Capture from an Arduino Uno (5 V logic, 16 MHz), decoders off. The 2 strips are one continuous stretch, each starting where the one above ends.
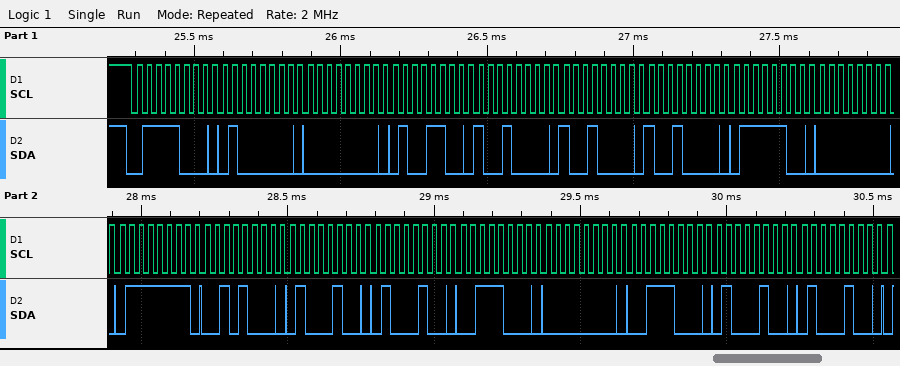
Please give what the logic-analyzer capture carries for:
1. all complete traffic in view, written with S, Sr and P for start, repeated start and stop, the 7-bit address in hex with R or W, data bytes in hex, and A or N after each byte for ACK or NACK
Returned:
S 3CW A 40 A 00 A 4C A 90 A 90 A 90 A 7C A 00 A 7F A 28 A 44 A 44 A 38 A 00 A 38 A 44 A 44 A
